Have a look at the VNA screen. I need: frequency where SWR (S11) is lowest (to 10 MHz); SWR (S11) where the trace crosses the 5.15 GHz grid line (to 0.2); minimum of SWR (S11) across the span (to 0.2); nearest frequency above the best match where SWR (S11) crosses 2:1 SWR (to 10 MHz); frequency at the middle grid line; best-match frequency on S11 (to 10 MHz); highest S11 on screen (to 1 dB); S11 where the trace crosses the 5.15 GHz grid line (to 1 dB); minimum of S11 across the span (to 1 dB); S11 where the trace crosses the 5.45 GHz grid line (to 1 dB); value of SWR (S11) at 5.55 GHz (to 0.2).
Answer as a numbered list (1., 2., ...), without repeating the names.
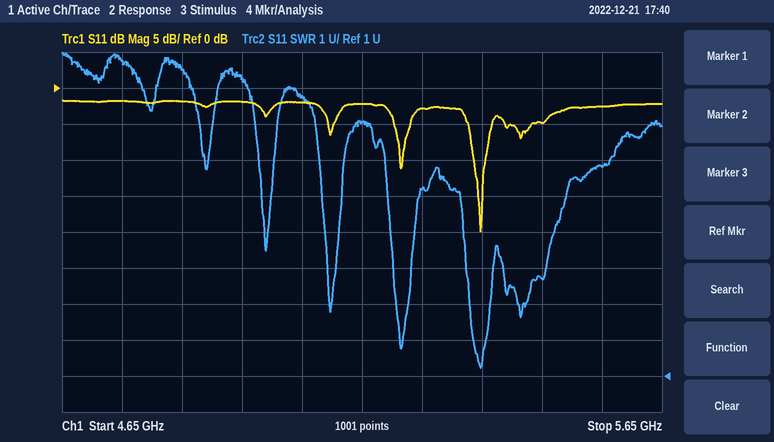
1. 5.35 GHz
2. 8.0
3. 1.2
4. 5.36 GHz
5. 5.15 GHz
6. 5.35 GHz
7. -2 dB
8. -2 dB
9. -20 dB
10. -5 dB
11. 6.8
